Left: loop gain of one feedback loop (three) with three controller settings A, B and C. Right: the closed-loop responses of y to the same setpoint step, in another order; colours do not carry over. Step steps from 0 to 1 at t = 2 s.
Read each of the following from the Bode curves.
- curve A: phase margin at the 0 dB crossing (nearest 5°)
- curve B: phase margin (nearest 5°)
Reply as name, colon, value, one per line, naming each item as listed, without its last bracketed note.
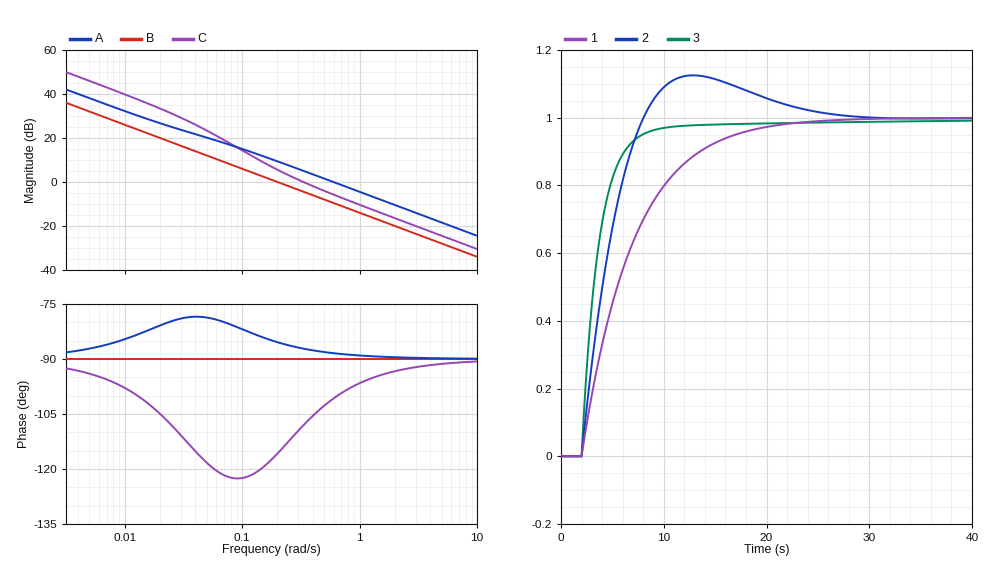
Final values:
curve A: phase margin at the 0 dB crossing: 90°
curve B: phase margin: 90°
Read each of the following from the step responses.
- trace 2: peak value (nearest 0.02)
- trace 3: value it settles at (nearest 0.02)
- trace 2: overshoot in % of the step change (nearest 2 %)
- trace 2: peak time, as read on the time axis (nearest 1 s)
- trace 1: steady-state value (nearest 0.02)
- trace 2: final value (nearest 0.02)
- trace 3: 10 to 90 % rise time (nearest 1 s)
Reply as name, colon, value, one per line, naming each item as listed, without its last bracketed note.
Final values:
trace 2: peak value: 1.12
trace 3: value it settles at: 1.00
trace 2: overshoot in % of the step change: 12 %
trace 2: peak time, as read on the time axis: 13 s
trace 1: steady-state value: 1.00
trace 2: final value: 1.00
trace 3: 10 to 90 % rise time: 4 s
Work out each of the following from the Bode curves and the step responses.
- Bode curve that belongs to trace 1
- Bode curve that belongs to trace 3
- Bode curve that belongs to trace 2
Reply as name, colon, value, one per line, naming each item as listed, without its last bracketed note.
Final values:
Bode curve that belongs to trace 1: B
Bode curve that belongs to trace 3: A
Bode curve that belongs to trace 2: C
